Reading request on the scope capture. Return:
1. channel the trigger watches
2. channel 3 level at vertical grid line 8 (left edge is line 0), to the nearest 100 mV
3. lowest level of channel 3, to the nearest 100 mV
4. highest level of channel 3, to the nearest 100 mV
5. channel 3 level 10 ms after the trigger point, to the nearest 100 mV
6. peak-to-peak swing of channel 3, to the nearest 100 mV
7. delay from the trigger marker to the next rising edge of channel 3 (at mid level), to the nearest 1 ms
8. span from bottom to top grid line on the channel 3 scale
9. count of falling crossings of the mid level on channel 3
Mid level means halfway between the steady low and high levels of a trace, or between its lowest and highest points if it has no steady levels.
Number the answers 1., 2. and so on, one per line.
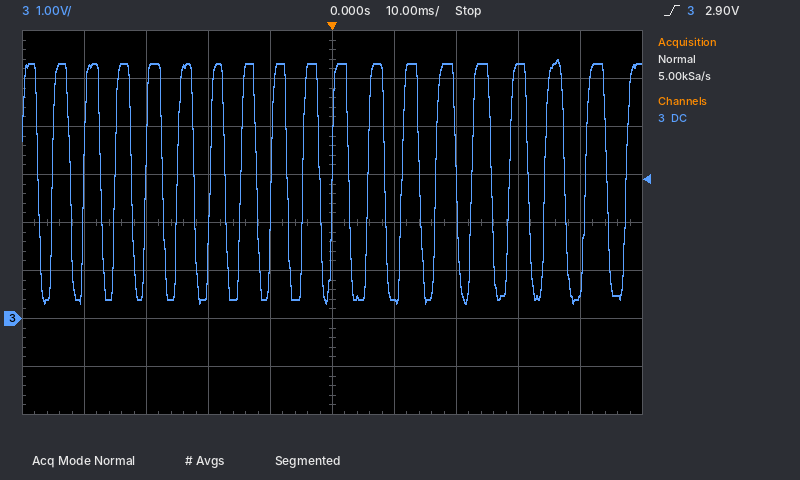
1. channel 3
2. 5.3 V
3. 300 mV
4. 5.4 V
5. 400 mV
6. 5.1 V
7. 6 ms
8. 8 V
9. 18
